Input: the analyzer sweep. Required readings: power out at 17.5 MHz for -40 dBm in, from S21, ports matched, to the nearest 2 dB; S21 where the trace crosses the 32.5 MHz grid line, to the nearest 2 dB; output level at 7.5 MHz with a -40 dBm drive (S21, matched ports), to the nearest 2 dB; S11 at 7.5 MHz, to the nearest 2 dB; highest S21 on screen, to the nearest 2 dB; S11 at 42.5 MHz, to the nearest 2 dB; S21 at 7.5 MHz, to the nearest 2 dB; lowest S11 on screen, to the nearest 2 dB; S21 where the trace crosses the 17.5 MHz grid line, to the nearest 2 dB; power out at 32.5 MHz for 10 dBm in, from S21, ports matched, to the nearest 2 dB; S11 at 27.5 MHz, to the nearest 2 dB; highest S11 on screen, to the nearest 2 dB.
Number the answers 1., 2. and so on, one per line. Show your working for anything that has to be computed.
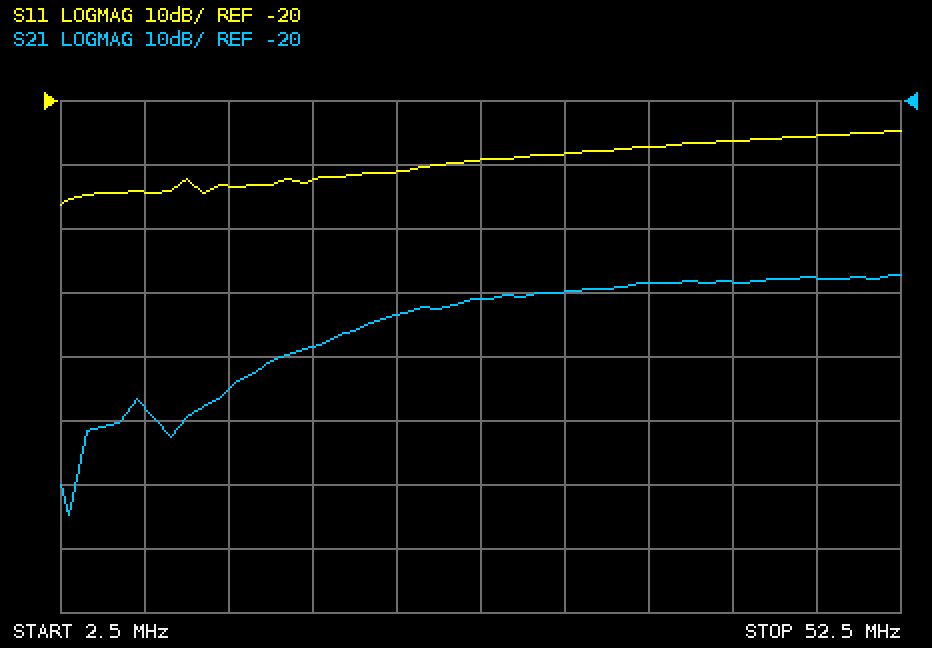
1. -40 dBm + (-58 dB) = -98 dBm
2. -50 dB
3. -40 dBm + (-68 dB) = -108 dBm
4. -34 dB
5. -48 dB
6. -26 dB
7. -68 dB
8. -36 dB
9. -58 dB
10. 10 dBm + (-50 dB) = -40 dBm
11. -30 dB
12. -24 dB
